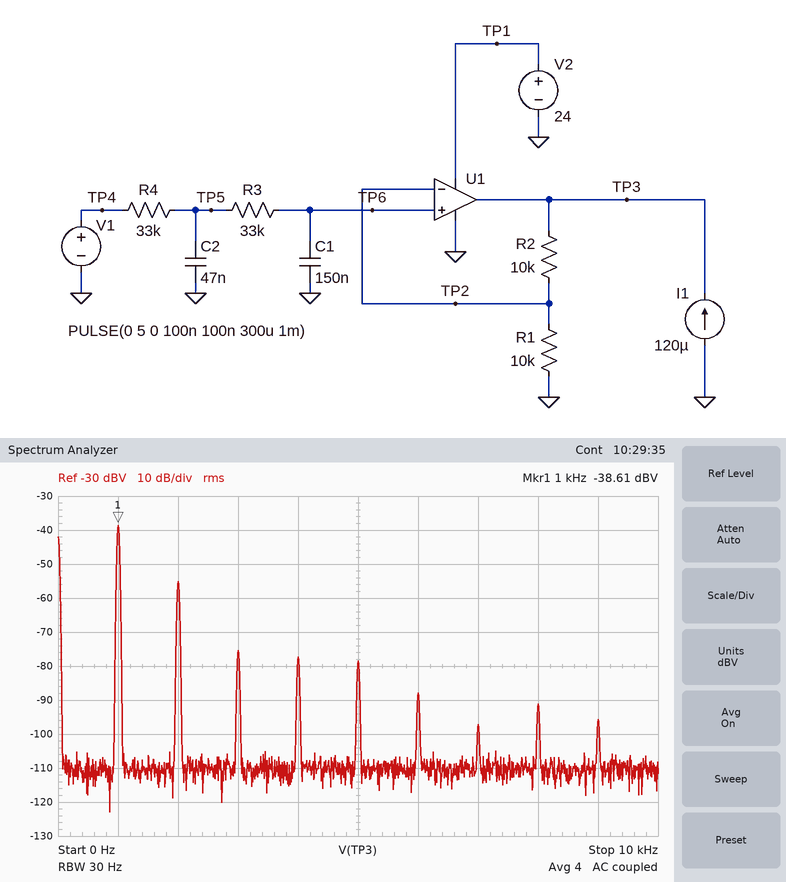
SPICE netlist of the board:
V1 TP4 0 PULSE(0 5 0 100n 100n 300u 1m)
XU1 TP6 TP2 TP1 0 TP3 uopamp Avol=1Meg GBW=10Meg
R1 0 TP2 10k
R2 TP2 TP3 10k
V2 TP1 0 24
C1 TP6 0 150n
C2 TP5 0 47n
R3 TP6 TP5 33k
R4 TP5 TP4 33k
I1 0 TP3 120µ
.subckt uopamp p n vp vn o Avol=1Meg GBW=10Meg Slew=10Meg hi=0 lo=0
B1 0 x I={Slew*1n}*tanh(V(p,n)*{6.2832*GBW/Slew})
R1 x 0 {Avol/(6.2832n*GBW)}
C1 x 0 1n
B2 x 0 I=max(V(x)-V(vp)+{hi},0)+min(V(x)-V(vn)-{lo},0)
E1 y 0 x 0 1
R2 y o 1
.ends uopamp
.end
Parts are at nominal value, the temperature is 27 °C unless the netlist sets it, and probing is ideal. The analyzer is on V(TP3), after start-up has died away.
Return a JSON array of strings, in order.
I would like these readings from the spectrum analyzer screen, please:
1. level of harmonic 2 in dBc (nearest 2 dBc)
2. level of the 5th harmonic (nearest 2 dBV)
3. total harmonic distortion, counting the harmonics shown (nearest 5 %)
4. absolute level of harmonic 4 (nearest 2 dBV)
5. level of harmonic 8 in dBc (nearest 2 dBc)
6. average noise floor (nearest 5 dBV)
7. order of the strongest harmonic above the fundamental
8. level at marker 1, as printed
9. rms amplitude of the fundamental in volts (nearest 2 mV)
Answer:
["-16 dBc", "-78 dBV", "15 %", "-78 dBV", "-52 dBc", "-110 dBV", "2", "-38.61 dBV", "12 mV"]
